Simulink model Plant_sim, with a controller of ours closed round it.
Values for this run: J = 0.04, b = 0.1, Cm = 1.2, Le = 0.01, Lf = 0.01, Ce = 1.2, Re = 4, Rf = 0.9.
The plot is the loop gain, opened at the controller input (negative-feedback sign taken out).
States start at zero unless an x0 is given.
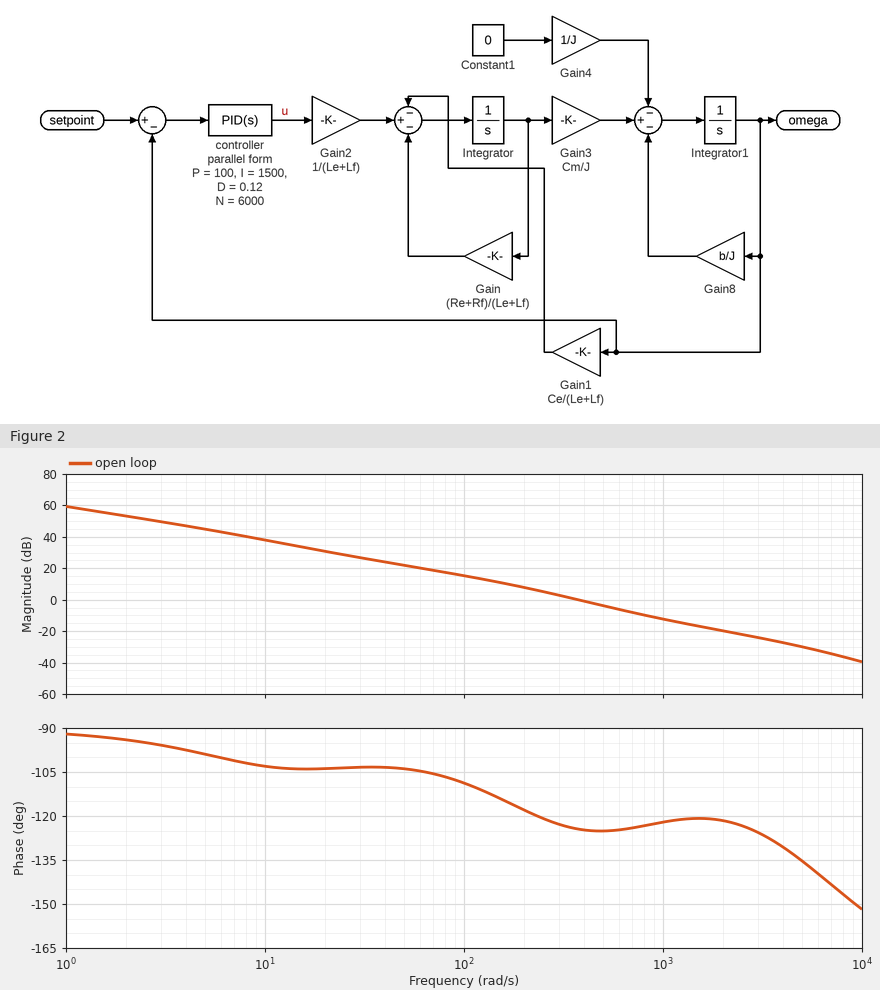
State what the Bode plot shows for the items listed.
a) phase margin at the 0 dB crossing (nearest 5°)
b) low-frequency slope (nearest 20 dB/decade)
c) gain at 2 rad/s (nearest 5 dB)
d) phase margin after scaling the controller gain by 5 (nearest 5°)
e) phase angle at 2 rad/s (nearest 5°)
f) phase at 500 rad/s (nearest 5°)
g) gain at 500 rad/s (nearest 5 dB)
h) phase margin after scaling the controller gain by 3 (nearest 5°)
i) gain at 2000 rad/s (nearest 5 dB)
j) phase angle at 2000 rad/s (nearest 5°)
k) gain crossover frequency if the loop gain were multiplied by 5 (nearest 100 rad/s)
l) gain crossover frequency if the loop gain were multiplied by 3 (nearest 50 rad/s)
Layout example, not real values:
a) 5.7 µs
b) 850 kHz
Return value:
a) 55°
b) -20 dB/decade
c) 55 dB
d) 60°
e) -95°
f) -125°
g) -5 dB
h) 55°
i) -20 dB
j) -120°
k) 1200 rad/s
l) 800 rad/s
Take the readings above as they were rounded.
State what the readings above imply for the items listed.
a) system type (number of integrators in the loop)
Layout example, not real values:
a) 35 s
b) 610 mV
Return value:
a) 1
